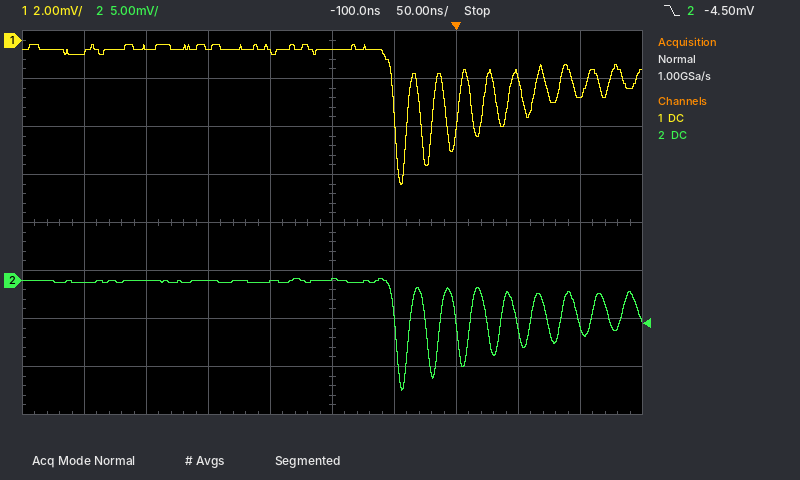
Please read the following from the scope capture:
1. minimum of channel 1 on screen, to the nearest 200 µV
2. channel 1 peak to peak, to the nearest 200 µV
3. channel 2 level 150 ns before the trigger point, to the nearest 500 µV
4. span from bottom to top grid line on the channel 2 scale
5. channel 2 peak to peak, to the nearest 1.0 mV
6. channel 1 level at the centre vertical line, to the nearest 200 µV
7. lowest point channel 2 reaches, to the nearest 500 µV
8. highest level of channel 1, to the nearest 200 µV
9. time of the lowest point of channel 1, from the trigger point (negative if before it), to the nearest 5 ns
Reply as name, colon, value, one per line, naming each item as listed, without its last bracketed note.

minimum of channel 1 on screen, to the nearest 200 µV: -6.0 mV
channel 1 peak to peak, to the nearest 200 µV: 5.8 mV
channel 2 level 150 ns before the trigger point, to the nearest 500 µV: 0.0 mV
span from bottom to top grid line on the channel 2 scale: 40 mV
channel 2 peak to peak, to the nearest 1.0 mV: 12.0 mV
channel 1 level at the centre vertical line, to the nearest 200 µV: -400 µV
lowest point channel 2 reaches, to the nearest 500 µV: -11.5 mV
highest level of channel 1, to the nearest 200 µV: -200 µV
time of the lowest point of channel 1, from the trigger point (negative if before it), to the nearest 5 ns: -45 ns
